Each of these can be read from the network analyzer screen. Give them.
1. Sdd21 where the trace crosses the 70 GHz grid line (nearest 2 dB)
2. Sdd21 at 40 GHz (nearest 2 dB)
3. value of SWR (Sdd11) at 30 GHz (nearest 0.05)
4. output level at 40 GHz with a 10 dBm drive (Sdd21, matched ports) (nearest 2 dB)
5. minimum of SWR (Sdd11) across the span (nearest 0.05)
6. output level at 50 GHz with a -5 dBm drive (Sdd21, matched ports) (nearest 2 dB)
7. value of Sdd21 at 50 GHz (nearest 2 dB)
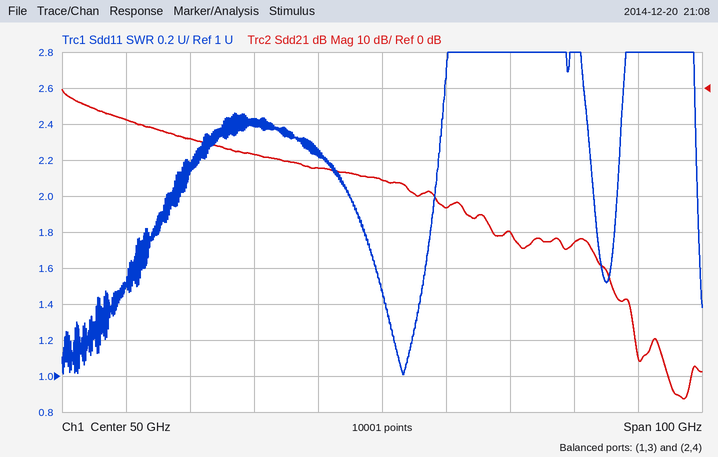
-40 dB
-22 dB
2.40
-12 dBm
1.00
-30 dBm
-26 dB
